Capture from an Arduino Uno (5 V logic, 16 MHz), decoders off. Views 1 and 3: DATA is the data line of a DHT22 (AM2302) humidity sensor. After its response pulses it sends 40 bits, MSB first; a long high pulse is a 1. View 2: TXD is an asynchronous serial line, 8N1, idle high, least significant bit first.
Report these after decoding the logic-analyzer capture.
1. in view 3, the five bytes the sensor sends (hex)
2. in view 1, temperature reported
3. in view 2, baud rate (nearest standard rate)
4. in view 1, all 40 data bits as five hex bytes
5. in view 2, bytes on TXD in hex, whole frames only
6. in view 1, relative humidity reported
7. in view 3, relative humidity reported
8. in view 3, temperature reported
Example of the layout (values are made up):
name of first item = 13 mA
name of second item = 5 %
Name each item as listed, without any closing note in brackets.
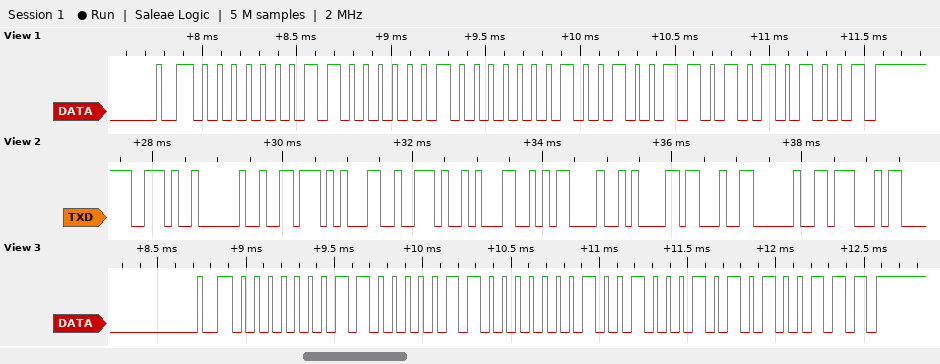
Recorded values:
in view 3, the five bytes the sensor sends = 01 83 01 22 A7
in view 1, temperature reported = 29.4 °C
in view 2, baud rate = 9600 baud
in view 1, all 40 data bits as five hex bytes = 01 81 01 26 A9
in view 2, bytes on TXD in hex, whole frames only = 2E 20 76 31 2E 31 0D 0A 23 20 47
in view 1, relative humidity reported = 38.5 %
in view 3, relative humidity reported = 38.7 %
in view 3, temperature reported = 29.0 °C
